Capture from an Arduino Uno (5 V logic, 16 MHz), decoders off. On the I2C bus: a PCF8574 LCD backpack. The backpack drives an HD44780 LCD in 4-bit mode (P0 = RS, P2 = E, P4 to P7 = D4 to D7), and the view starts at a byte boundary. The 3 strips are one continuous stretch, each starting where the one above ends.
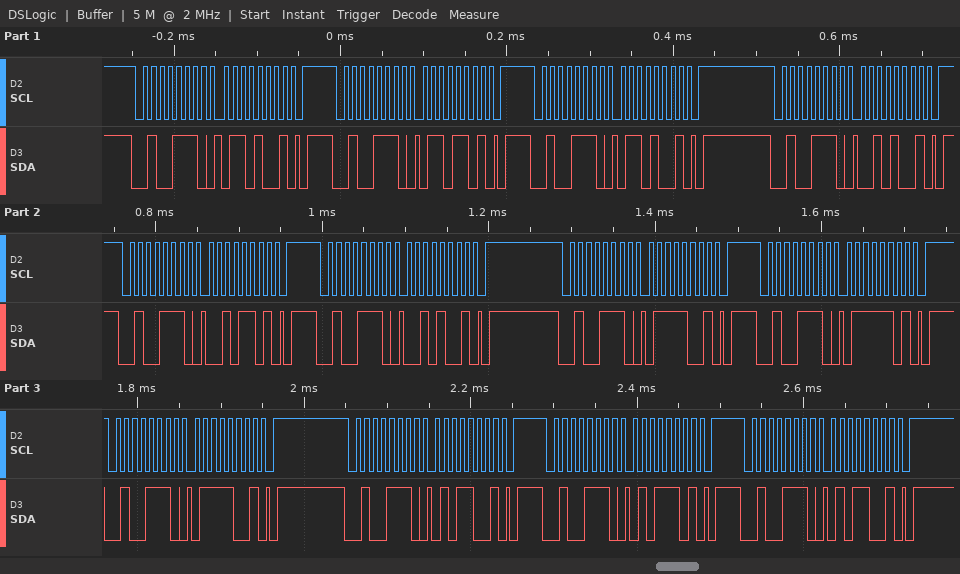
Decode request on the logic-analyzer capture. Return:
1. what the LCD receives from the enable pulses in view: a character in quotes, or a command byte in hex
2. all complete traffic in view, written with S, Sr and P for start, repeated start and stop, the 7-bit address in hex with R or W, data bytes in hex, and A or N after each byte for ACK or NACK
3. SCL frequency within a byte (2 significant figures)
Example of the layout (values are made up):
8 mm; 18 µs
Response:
'b' 'u'; S 27W A 69 A P S 27W A 6D A P S 27W A 69 A P S 27W A 29 A P S 27W A 2D A P S 27W A 29 A P S 27W A 79 A P S 27W A 7D A P S 27W A 79 A P S 27W A 59 A P S 27W A 5D A P S 27W A 59 A P; 100 kHz
